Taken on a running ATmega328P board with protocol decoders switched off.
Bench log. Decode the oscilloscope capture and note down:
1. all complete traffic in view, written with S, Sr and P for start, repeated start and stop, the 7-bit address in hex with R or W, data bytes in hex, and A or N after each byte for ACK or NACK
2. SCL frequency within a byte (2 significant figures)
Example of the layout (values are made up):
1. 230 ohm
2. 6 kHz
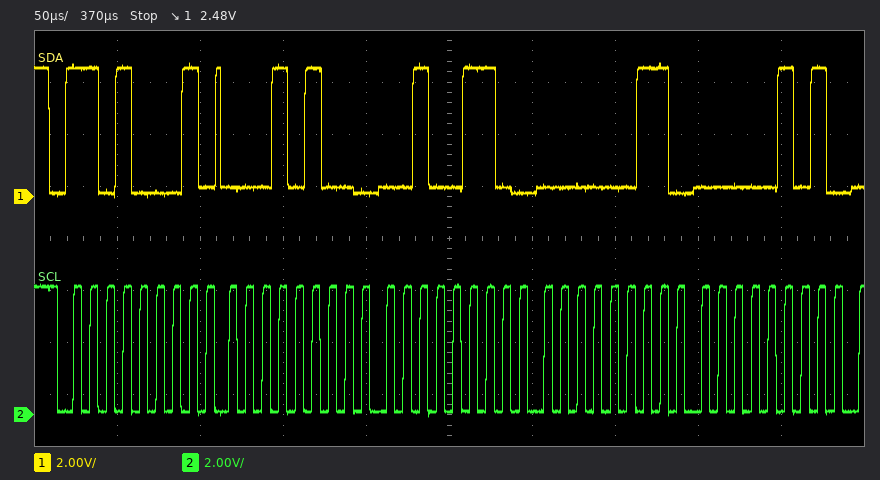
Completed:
1. S 68R A 14 A 26 A 03 A 05 A
2. 100 kHz
